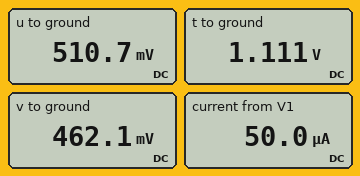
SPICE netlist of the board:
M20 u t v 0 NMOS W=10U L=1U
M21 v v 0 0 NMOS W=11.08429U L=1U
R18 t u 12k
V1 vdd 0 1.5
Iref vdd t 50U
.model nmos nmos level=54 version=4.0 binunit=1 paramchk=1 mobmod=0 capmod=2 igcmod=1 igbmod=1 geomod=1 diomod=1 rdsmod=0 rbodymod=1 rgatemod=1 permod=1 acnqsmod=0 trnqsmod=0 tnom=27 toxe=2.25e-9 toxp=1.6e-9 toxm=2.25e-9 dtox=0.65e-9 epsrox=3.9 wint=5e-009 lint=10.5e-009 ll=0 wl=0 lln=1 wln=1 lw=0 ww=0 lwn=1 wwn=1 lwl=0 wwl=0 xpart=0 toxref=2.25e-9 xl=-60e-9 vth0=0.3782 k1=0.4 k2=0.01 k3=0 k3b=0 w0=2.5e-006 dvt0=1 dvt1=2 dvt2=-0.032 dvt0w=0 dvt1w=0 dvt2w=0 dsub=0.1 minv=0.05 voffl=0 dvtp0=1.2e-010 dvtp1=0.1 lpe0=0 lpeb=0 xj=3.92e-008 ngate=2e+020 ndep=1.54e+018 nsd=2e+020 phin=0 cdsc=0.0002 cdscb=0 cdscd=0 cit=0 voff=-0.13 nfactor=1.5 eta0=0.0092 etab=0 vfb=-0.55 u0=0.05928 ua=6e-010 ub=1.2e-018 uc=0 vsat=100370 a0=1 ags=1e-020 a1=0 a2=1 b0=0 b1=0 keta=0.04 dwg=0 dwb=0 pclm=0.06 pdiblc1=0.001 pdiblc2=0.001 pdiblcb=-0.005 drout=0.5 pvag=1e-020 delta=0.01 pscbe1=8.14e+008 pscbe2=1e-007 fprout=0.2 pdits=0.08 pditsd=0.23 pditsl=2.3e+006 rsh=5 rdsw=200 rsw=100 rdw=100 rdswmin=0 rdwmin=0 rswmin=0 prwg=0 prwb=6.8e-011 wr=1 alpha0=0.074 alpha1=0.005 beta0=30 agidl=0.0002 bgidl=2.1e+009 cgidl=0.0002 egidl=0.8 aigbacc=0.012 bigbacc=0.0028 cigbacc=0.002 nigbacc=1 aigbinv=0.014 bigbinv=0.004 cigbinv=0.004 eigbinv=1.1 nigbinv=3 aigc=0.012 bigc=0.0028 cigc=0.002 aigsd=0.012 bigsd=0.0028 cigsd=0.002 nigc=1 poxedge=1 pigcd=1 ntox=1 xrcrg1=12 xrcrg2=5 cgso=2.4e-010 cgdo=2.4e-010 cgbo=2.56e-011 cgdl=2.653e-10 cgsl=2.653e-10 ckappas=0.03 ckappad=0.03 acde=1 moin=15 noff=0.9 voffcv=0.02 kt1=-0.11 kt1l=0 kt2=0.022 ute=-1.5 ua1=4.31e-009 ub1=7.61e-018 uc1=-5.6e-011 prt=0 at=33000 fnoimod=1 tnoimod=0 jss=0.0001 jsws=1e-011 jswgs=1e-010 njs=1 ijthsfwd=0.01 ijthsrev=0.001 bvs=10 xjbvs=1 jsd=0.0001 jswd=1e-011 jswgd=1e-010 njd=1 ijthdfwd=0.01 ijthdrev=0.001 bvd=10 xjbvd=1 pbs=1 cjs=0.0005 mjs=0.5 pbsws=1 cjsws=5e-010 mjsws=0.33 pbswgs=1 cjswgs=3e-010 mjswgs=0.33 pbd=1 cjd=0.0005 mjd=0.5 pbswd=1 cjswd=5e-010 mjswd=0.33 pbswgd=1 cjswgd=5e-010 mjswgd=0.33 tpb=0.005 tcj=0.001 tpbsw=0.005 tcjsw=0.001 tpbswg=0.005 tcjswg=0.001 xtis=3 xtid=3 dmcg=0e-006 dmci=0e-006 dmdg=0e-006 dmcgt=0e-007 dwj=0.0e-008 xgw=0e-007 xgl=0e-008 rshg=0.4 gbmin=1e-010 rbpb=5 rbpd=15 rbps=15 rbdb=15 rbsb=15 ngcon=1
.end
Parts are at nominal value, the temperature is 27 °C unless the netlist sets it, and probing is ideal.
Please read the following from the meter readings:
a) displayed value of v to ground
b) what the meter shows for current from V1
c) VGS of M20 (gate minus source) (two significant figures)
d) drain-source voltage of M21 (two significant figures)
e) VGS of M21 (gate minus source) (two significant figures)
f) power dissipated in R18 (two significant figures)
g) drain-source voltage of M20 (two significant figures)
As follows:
462.1 mV
50.0 µA
650 mV
460 mV
460 mV
30 µW
49 mV
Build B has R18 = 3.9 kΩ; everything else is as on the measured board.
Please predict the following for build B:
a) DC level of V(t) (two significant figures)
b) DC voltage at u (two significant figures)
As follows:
1.0 V
840 mV
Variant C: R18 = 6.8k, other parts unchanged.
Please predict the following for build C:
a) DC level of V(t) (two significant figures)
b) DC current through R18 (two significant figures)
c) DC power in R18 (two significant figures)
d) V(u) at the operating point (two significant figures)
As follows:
1.0 V
50 µA
17 µW
690 mV
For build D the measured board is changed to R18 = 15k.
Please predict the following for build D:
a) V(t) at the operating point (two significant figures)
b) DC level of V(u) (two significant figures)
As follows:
1.2 V
490 mV
